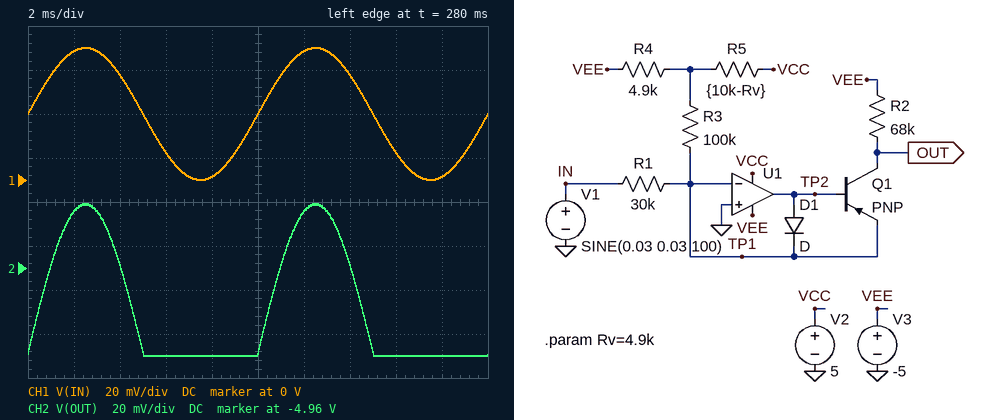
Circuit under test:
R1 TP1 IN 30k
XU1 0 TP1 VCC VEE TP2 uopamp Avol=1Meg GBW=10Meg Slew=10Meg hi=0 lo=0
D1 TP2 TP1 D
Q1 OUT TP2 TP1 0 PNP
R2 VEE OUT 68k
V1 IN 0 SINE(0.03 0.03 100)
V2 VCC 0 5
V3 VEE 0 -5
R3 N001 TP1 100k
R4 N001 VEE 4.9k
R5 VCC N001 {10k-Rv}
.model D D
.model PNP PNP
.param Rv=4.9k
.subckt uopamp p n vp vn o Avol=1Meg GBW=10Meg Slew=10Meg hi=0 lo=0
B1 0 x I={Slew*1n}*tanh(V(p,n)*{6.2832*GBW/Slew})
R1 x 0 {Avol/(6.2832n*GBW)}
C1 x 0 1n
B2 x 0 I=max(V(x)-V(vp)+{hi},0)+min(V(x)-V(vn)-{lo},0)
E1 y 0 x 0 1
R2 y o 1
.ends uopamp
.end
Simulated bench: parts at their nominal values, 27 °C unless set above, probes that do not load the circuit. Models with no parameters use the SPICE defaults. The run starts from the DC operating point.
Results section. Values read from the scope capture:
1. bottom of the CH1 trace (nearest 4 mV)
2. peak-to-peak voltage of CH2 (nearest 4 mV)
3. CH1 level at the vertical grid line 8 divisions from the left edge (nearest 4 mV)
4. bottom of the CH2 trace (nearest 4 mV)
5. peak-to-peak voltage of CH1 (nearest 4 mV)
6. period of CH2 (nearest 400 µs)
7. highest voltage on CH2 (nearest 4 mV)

0 V
68 mV
12 mV
-5.000 V
60 mV
10.0 ms
-4.932 V
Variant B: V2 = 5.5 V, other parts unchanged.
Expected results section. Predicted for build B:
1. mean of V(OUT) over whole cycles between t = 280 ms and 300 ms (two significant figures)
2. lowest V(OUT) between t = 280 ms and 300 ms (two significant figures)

-4.8 V
-4.9 V
